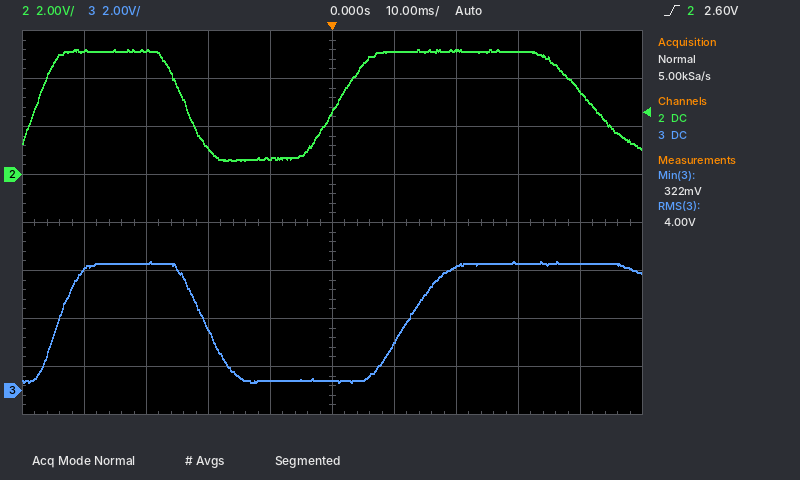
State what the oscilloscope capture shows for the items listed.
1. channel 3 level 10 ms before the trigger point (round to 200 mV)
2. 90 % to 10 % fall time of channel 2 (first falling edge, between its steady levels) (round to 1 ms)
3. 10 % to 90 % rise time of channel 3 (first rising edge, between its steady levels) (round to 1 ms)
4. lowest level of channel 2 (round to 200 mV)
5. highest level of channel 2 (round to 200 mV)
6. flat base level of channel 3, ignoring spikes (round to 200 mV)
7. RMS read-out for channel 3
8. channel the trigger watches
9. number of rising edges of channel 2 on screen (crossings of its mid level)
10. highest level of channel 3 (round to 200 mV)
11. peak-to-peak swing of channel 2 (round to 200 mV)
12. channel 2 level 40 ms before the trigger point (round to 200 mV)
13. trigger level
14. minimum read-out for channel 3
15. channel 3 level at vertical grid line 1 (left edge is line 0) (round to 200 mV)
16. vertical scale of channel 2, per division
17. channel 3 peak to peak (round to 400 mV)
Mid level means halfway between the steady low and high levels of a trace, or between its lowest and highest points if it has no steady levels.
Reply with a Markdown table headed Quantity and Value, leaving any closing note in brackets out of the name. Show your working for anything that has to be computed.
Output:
| Quantity | Value |
|---|---|
| channel 3 level 10 ms before the trigger point | 400 mV |
| 90 % to 10 % fall time of channel 2 (first falling edge, between its steady levels) | 7 ms |
| 10 % to 90 % rise time of channel 3 (first rising edge, between its steady levels) | 6 ms |
| lowest level of channel 2 | 600 mV |
| highest level of channel 2 | 5.2 V |
| flat base level of channel 3, ignoring spikes | 400 mV |
| RMS read-out for channel 3 | 4.00 V |
| channel the trigger watches | channel 2 |
| number of rising edges of channel 2 on screen | 2 |
| highest level of channel 3 | 5.4 V |
| peak-to-peak swing of channel 2 | 5.2 V − (600 mV) = 4.6 V |
| channel 2 level 40 ms before the trigger point | 5.2 V |
| trigger level | 2.60 V |
| minimum read-out for channel 3 | 322 mV |
| channel 3 level at vertical grid line 1 (left edge is line 0) | 5.0 V |
| vertical scale of channel 2, per division | 2 V |
| channel 3 peak to peak | 5.2 V |
